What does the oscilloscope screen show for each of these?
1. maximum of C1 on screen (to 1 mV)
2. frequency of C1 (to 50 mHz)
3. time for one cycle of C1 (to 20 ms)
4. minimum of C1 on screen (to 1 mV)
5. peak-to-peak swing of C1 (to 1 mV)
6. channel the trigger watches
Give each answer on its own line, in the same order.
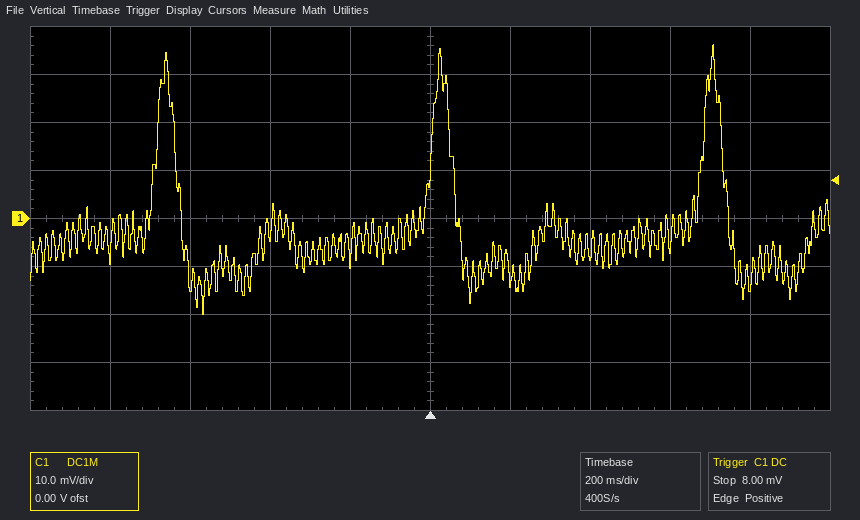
36 mV
1.45 Hz
680 ms
-20 mV
56 mV
C1
